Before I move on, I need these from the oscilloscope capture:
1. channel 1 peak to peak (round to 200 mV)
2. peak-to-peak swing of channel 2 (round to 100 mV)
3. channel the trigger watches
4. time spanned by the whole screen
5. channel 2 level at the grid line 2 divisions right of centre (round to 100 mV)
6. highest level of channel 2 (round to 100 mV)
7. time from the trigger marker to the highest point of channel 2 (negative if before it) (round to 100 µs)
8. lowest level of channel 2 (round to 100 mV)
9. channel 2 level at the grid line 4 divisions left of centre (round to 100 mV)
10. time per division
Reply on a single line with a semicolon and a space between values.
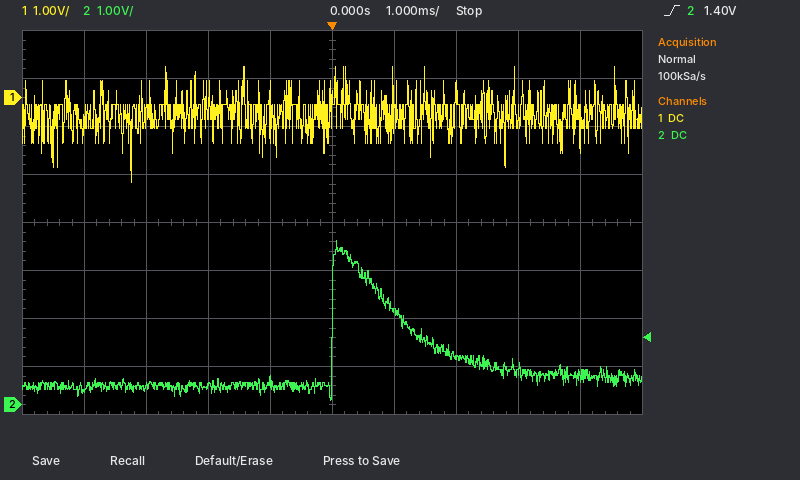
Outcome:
2.4 V; 3.3 V; channel 2; 10 ms; 1.0 V; 3.4 V; +100 µs; 100 mV; 300 mV; 1 ms
